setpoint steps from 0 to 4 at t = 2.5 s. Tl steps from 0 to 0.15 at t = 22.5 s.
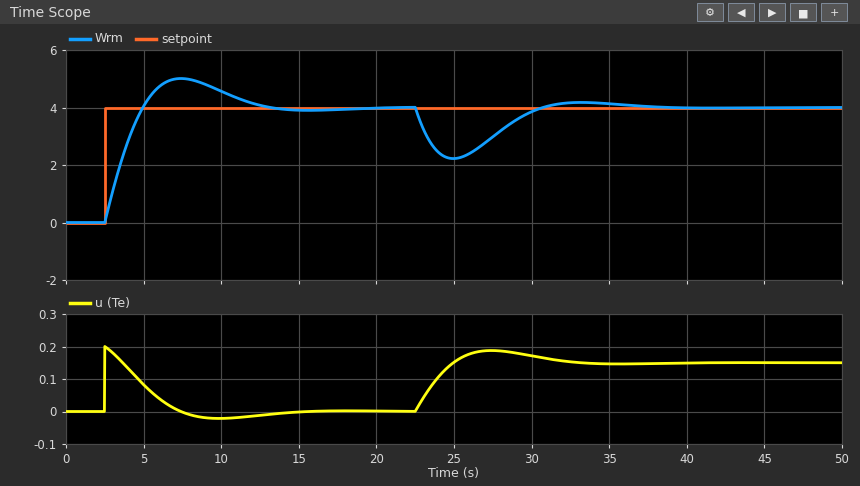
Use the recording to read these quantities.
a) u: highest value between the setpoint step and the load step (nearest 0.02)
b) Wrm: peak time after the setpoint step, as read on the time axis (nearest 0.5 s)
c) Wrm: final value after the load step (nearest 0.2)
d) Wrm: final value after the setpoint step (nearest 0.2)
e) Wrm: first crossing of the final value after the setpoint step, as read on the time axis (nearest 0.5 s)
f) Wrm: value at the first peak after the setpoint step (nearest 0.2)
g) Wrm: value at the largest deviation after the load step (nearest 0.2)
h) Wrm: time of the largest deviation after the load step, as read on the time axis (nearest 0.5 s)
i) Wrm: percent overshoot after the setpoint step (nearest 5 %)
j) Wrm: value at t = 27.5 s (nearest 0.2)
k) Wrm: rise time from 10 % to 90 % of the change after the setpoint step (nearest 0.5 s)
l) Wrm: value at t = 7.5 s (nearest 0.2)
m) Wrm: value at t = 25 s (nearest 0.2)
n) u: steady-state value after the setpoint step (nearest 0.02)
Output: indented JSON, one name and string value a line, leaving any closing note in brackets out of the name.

{
  "u: highest value between the setpoint step and the load step": "0.20",
  "Wrm: peak time after the setpoint step, as read on the time axis": "7.5 s",
  "Wrm: final value after the load step": "4.0",
  "Wrm: final value after the setpoint step": "4.0",
  "Wrm: first crossing of the final value after the setpoint step, as read on the time axis": "5.0 s",
  "Wrm: value at the first peak after the setpoint step": "5.0",
  "Wrm: value at the largest deviation after the load step": "2.2",
  "Wrm: time of the largest deviation after the load step, as read on the time axis": "25.0 s",
  "Wrm: percent overshoot after the setpoint step": "25 %",
  "Wrm: value at t = 27.5 s": "3.0",
  "Wrm: rise time from 10 % to 90 % of the change after the setpoint step": "2.0 s",
  "Wrm: value at t = 7.5 s": "5.0",
  "Wrm: value at t = 25 s": "2.2",
  "u: steady-state value after the setpoint step": "0.00"
}
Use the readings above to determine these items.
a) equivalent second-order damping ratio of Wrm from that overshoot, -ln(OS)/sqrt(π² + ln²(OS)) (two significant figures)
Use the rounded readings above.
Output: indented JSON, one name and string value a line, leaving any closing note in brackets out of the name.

{
  "equivalent second-order damping ratio of Wrm from that overshoot, -ln(OS)/sqrt(π² + ln²(OS))": "0.40"
}
